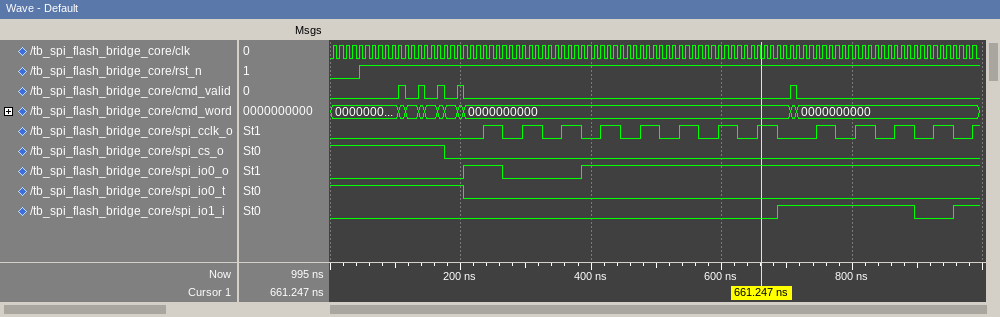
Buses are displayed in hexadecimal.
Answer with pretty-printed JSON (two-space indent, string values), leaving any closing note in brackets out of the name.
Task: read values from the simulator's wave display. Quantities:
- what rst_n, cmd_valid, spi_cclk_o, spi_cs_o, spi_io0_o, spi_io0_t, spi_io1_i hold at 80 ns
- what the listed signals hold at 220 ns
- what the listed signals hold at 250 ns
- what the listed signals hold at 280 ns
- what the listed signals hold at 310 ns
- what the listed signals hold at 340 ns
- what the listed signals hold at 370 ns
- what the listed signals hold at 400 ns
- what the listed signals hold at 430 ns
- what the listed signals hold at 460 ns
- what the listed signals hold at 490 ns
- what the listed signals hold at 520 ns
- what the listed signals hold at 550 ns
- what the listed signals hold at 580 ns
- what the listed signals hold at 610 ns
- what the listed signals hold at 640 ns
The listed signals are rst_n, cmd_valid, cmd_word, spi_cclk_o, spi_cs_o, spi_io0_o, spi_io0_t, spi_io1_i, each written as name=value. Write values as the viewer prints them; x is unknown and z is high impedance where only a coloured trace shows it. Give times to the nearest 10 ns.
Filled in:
{
  "what rst_n, cmd_valid, spi_cclk_o, spi_cs_o, spi_io0_o, spi_io0_t, spi_io1_i hold at 80 ns": "rst_n=1, cmd_valid=0, spi_cclk_o=0, spi_cs_o=1, spi_io0_o=0, spi_io0_t=1, spi_io1_i=0",
  "what the listed signals hold at 220 ns": "rst_n=1, cmd_valid=0, cmd_word=0000000000, spi_cclk_o=0, spi_cs_o=0, spi_io0_o=1, spi_io0_t=0, spi_io1_i=0",
  "what the listed signals hold at 250 ns": "rst_n=1, cmd_valid=0, cmd_word=0000000000, spi_cclk_o=1, spi_cs_o=0, spi_io0_o=1, spi_io0_t=0, spi_io1_i=0",
  "what the listed signals hold at 280 ns": "rst_n=1, cmd_valid=0, cmd_word=0000000000, spi_cclk_o=0, spi_cs_o=0, spi_io0_o=0, spi_io0_t=0, spi_io1_i=0",
  "what the listed signals hold at 310 ns": "rst_n=1, cmd_valid=0, cmd_word=0000000000, spi_cclk_o=1, spi_cs_o=0, spi_io0_o=0, spi_io0_t=0, spi_io1_i=0",
  "what the listed signals hold at 340 ns": "rst_n=1, cmd_valid=0, cmd_word=0000000000, spi_cclk_o=0, spi_cs_o=0, spi_io0_o=0, spi_io0_t=0, spi_io1_i=0",
  "what the listed signals hold at 370 ns": "rst_n=1, cmd_valid=0, cmd_word=0000000000, spi_cclk_o=1, spi_cs_o=0, spi_io0_o=0, spi_io0_t=0, spi_io1_i=0",
  "what the listed signals hold at 400 ns": "rst_n=1, cmd_valid=0, cmd_word=0000000000, spi_cclk_o=0, spi_cs_o=0, spi_io0_o=1, spi_io0_t=0, spi_io1_i=0",
  "what the listed signals hold at 430 ns": "rst_n=1, cmd_valid=0, cmd_word=0000000000, spi_cclk_o=1, spi_cs_o=0, spi_io0_o=1, spi_io0_t=0, spi_io1_i=0",
  "what the listed signals hold at 460 ns": "rst_n=1, cmd_valid=0, cmd_word=0000000000, spi_cclk_o=0, spi_cs_o=0, spi_io0_o=1, spi_io0_t=0, spi_io1_i=0",
  "what the listed signals hold at 490 ns": "rst_n=1, cmd_valid=0, cmd_word=0000000000, spi_cclk_o=1, spi_cs_o=0, spi_io0_o=1, spi_io0_t=0, spi_io1_i=0",
  "what the listed signals hold at 520 ns": "rst_n=1, cmd_valid=0, cmd_word=0000000000, spi_cclk_o=0, spi_cs_o=0, spi_io0_o=1, spi_io0_t=0, spi_io1_i=0",
  "what the listed signals hold at 550 ns": "rst_n=1, cmd_valid=0, cmd_word=0000000000, spi_cclk_o=1, spi_cs_o=0, spi_io0_o=1, spi_io0_t=0, spi_io1_i=0",
  "what the listed signals hold at 580 ns": "rst_n=1, cmd_valid=0, cmd_word=0000000000, spi_cclk_o=0, spi_cs_o=0, spi_io0_o=1, spi_io0_t=0, spi_io1_i=0",
  "what the listed signals hold at 610 ns": "rst_n=1, cmd_valid=0, cmd_word=0000000000, spi_cclk_o=1, spi_cs_o=0, spi_io0_o=1, spi_io0_t=0, spi_io1_i=0",
  "what the listed signals hold at 640 ns": "rst_n=1, cmd_valid=0, cmd_word=0000000000, spi_cclk_o=0, spi_cs_o=0, spi_io0_o=1, spi_io0_t=0, spi_io1_i=0"
}
